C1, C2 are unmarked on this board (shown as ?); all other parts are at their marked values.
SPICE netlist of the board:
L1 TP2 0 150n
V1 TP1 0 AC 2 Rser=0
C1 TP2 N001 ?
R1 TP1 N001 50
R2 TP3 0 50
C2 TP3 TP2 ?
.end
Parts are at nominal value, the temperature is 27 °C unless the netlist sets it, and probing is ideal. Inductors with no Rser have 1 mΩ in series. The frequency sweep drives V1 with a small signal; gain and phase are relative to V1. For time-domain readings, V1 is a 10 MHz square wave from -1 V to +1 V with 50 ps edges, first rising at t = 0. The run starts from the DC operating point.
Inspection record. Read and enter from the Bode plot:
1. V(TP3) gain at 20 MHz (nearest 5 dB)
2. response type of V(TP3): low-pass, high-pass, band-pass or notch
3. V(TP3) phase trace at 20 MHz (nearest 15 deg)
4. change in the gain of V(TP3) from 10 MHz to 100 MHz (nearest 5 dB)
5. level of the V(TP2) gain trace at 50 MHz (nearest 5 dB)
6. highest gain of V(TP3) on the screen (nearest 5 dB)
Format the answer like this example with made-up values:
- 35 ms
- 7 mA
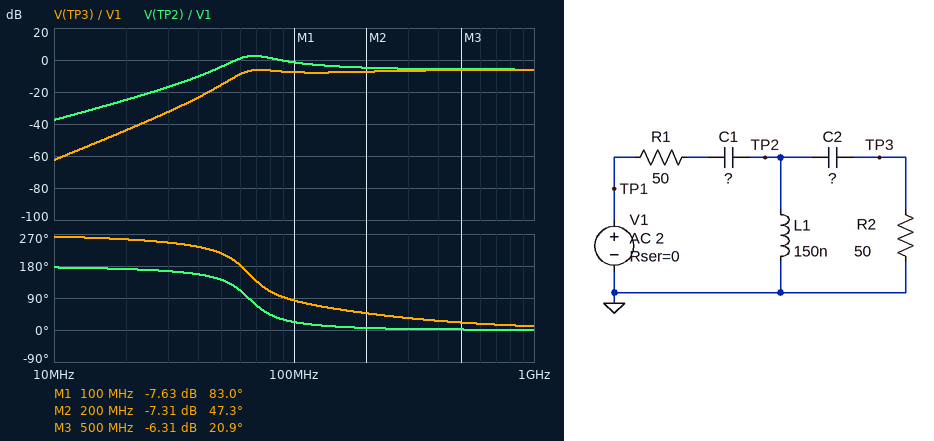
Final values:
- -45 dB
- high-pass
- 255 deg
- 55 dB
- -5 dB
- -5 dB
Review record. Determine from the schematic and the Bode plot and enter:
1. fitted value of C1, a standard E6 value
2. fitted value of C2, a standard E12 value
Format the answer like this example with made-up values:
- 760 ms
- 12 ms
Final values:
- 22 pF
- 18 pF
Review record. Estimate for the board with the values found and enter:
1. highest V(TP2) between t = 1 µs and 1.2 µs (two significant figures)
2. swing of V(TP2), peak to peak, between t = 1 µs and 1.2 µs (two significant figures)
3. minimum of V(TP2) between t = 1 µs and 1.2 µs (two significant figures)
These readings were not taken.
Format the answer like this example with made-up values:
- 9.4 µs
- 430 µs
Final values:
- 990 mV
- 2.0 V
- -990 mV
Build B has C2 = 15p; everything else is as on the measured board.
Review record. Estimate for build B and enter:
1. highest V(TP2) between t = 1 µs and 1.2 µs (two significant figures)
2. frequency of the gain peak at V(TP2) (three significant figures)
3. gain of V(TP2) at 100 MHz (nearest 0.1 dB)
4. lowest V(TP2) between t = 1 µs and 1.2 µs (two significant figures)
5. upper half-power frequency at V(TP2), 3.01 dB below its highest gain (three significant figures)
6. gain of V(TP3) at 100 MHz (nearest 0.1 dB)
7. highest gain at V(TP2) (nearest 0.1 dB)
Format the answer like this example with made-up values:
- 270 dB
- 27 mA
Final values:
- 1.0 V
- 70.6 MHz
- -0.5 dB
- -1.0 V
- 93.0 MHz
- -7.9 dB
- 3.4 dB
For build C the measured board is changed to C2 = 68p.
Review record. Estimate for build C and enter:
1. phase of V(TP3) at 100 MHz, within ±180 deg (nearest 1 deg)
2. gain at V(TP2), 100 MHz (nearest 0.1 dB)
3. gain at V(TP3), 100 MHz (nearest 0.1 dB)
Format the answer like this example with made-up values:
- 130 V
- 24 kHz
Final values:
- 65 deg
- -6.4 dB
- -7.3 dB
